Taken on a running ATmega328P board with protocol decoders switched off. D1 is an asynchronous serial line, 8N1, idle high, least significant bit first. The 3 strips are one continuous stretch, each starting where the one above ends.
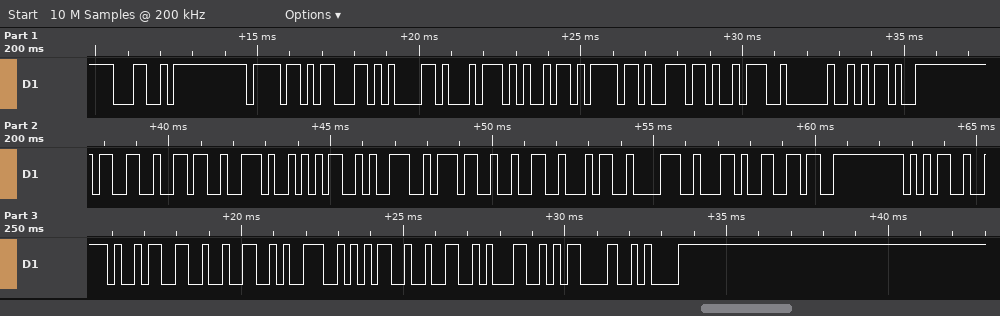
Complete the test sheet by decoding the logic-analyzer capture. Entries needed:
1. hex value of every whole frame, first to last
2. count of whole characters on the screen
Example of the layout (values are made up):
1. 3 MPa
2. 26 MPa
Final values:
1. 0x4C 0x6F 0x63 0x61 0x74 0x69 0x6F 0x6E 0x3A 0x20 0x2D 0x33 0x36 0x2E 0x35 0x39 0x37 0x32 0x34 0x38 0x2C 0x36 0x35 0x2E 0x33 0x32 0x39 0x35 0x32 0x31 0x0D 0x0A
2. 32
